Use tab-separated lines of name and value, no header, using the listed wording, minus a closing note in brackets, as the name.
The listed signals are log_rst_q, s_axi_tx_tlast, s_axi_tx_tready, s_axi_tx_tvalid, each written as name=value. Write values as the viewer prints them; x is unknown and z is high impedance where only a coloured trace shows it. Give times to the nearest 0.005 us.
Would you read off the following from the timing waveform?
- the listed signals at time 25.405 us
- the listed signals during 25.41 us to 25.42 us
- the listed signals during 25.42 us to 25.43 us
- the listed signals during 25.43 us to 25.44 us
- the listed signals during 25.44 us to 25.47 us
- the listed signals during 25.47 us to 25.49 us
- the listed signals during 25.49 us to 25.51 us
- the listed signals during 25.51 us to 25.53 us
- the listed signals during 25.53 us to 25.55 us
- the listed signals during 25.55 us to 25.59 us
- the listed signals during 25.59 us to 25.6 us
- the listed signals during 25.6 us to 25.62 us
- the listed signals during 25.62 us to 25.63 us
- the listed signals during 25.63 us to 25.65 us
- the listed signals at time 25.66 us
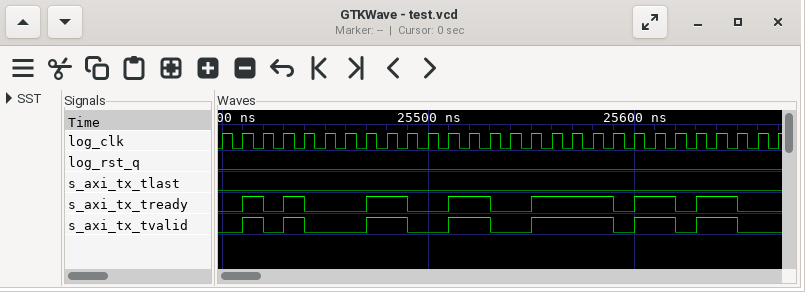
the listed signals at time 25.405 us	log_rst_q=0, s_axi_tx_tlast=0, s_axi_tx_tready=0, s_axi_tx_tvalid=0
the listed signals during 25.41 us to 25.42 us	log_rst_q=0, s_axi_tx_tlast=0, s_axi_tx_tready=1, s_axi_tx_tvalid=1
the listed signals during 25.42 us to 25.43 us	log_rst_q=0, s_axi_tx_tlast=0, s_axi_tx_tready=0, s_axi_tx_tvalid=0
the listed signals during 25.43 us to 25.44 us	log_rst_q=0, s_axi_tx_tlast=0, s_axi_tx_tready=1, s_axi_tx_tvalid=1
the listed signals during 25.44 us to 25.47 us	log_rst_q=0, s_axi_tx_tlast=0, s_axi_tx_tready=0, s_axi_tx_tvalid=0
the listed signals during 25.47 us to 25.49 us	log_rst_q=0, s_axi_tx_tlast=0, s_axi_tx_tready=1, s_axi_tx_tvalid=1
the listed signals during 25.49 us to 25.51 us	log_rst_q=0, s_axi_tx_tlast=0, s_axi_tx_tready=0, s_axi_tx_tvalid=0
the listed signals during 25.51 us to 25.53 us	log_rst_q=0, s_axi_tx_tlast=0, s_axi_tx_tready=1, s_axi_tx_tvalid=1
the listed signals during 25.53 us to 25.55 us	log_rst_q=0, s_axi_tx_tlast=0, s_axi_tx_tready=0, s_axi_tx_tvalid=0
the listed signals during 25.55 us to 25.59 us	log_rst_q=0, s_axi_tx_tlast=0, s_axi_tx_tready=1, s_axi_tx_tvalid=1
the listed signals during 25.59 us to 25.6 us	log_rst_q=0, s_axi_tx_tlast=0, s_axi_tx_tready=0, s_axi_tx_tvalid=0
the listed signals during 25.6 us to 25.62 us	log_rst_q=0, s_axi_tx_tlast=0, s_axi_tx_tready=1, s_axi_tx_tvalid=1
the listed signals during 25.62 us to 25.63 us	log_rst_q=0, s_axi_tx_tlast=0, s_axi_tx_tready=0, s_axi_tx_tvalid=0
the listed signals during 25.63 us to 25.65 us	log_rst_q=0, s_axi_tx_tlast=0, s_axi_tx_tready=1, s_axi_tx_tvalid=1
the listed signals at time 25.66 us	log_rst_q=0, s_axi_tx_tlast=0, s_axi_tx_tready=0, s_axi_tx_tvalid=0
